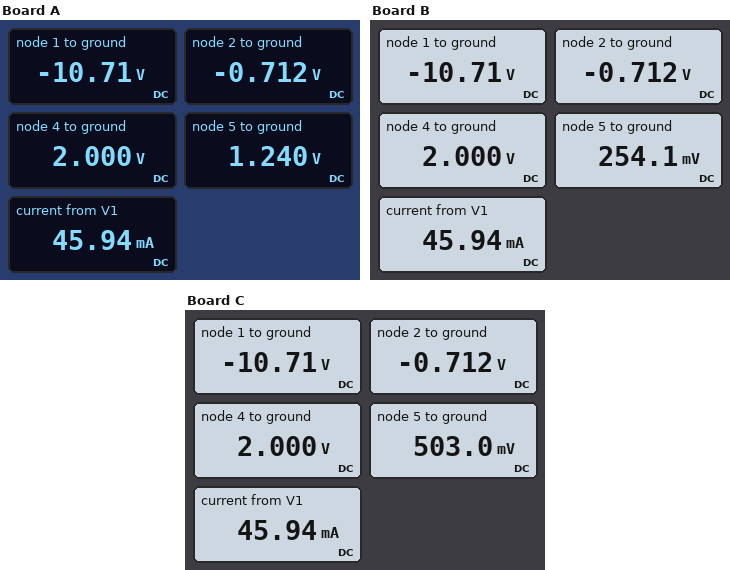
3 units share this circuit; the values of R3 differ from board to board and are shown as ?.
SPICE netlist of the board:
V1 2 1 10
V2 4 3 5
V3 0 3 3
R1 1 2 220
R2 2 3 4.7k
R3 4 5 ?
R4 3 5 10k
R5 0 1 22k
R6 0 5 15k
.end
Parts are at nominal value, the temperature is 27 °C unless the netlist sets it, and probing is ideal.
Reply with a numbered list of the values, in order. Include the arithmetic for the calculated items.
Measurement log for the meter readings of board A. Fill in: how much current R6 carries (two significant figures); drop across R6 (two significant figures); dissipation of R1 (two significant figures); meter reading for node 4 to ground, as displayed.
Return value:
1. (1.24 V) / 15 kΩ = 83 µA
2. 1.24 V = 1.2 V
3. (-712 mV - (-10.71 V))^2 / 220 Ω = 450 mW
4. 2.000 V
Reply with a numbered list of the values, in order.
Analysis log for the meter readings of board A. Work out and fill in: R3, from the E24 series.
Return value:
1. 1.5 kΩ
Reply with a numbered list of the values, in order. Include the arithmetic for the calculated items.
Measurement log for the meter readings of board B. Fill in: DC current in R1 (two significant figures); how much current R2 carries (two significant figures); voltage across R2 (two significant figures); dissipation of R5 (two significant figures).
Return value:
1. (-712 mV - (-10.71 V)) / 220 Ω = 45 mA
2. (-712 mV - (-3 V)) / 4.7 kΩ = 490 µA
3. -712 mV - (-3 V) = 2.3 V
4. (0 V - (-10.71 V))^2 / 22 kΩ = 5.2 mW
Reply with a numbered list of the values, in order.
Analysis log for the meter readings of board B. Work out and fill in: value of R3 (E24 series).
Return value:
1. 5.1 kΩ
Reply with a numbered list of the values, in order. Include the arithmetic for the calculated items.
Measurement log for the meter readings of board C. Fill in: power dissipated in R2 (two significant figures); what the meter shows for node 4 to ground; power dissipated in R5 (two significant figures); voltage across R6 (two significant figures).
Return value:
1. (-712 mV - (-3 V))^2 / 4.7 kΩ = 1.1 mW
2. 2.000 V
3. (0 V - (-10.71 V))^2 / 22 kΩ = 5.2 mW
4. 503 mV = 500 mV
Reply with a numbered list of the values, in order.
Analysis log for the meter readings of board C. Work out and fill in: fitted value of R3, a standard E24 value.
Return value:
1. 3.9 kΩ
